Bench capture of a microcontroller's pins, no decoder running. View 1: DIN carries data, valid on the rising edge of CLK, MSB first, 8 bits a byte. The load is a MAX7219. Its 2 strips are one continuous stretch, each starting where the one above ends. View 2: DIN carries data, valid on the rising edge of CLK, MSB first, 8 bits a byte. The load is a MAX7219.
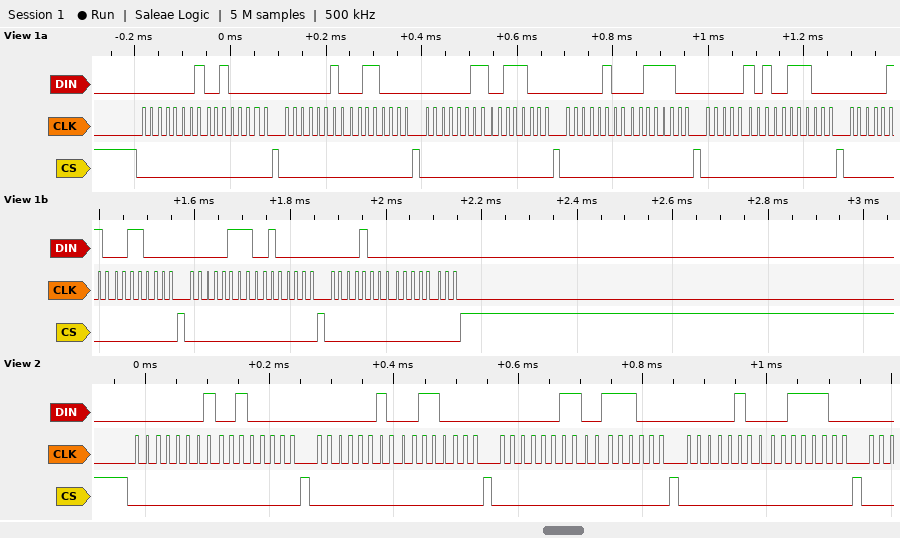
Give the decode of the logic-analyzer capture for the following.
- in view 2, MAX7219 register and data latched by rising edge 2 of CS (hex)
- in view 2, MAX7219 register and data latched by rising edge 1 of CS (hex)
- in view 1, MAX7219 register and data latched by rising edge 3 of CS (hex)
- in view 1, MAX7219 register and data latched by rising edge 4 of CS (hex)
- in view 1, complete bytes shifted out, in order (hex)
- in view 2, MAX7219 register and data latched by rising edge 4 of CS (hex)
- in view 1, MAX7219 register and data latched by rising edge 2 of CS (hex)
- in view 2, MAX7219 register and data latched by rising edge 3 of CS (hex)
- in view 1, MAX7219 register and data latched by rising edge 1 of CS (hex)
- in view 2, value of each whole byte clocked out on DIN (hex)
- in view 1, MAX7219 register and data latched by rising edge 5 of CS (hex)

register 0x2, data 0x30
register 0x1, data 0x20
register 0x3, data 0x38
register 0x4, data 0x3C
01 20 02 30 03 38 04 3C 05 38 06 30 07 20 08 00
register 0x4, data 0x3C
register 0x2, data 0x30
register 0x3, data 0x38
register 0x1, data 0x20
01 20 02 30 03 38 04 3C
register 0x5, data 0x38
